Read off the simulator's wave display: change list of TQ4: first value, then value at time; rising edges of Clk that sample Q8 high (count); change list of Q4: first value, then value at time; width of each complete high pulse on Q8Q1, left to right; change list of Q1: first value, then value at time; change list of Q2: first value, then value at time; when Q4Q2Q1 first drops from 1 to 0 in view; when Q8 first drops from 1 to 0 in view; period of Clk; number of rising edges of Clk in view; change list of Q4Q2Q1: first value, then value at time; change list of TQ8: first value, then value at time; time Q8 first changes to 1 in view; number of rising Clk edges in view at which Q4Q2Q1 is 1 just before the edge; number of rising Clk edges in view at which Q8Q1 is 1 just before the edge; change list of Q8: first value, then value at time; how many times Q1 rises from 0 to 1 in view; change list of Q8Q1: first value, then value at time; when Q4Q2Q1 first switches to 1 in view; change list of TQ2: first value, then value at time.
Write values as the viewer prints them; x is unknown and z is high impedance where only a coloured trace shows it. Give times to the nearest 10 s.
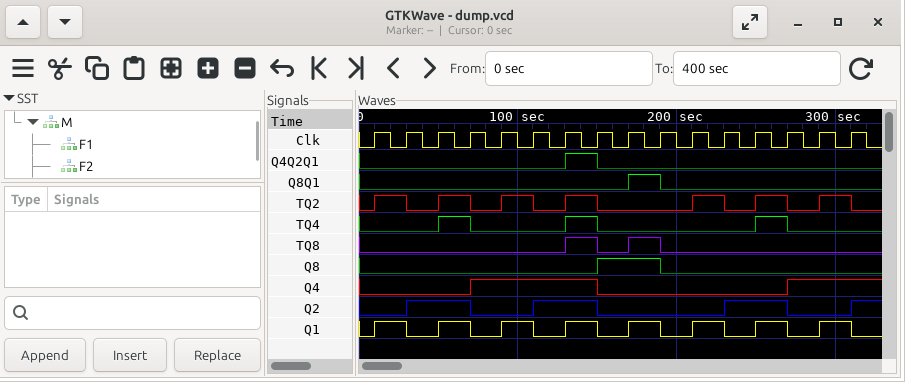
0, 1 at 50 s, 0 at 70 s, 1 at 130 s, 0 at 150 s, 1 at 250 s, 0 at 270 s
2
0, 1 at 70 s, 0 at 150 s, 1 at 270 s
20 s
0, 1 at 10 s, 0 at 30 s, 1 at 50 s, 0 at 70 s, 1 at 90 s, 0 at 110 s, 1 at 130 s, 0 at 150 s, 1 at 170 s, 0 at 190 s, 1 at 210 s, 0 at 230 s, 1 at 250 s, 0 at 270 s, 1 at 290 s, 0 at 310 s
0, 1 at 30 s, 0 at 70 s, 1 at 110 s, 0 at 150 s, 1 at 230 s, 0 at 270 s, 1 at 310 s
150 s
190 s
20 s
16
0, 1 at 130 s, 0 at 150 s
0, 1 at 130 s, 0 at 150 s, 1 at 170 s, 0 at 190 s
150 s
1
1
0, 1 at 150 s, 0 at 190 s
8
0, 1 at 170 s, 0 at 190 s
130 s
0, 1 at 10 s, 0 at 30 s, 1 at 50 s, 0 at 70 s, 1 at 90 s, 0 at 110 s, 1 at 130 s, 0 at 150 s, 1 at 210 s, 0 at 230 s, 1 at 250 s, 0 at 270 s, 1 at 290 s, 0 at 310 s
